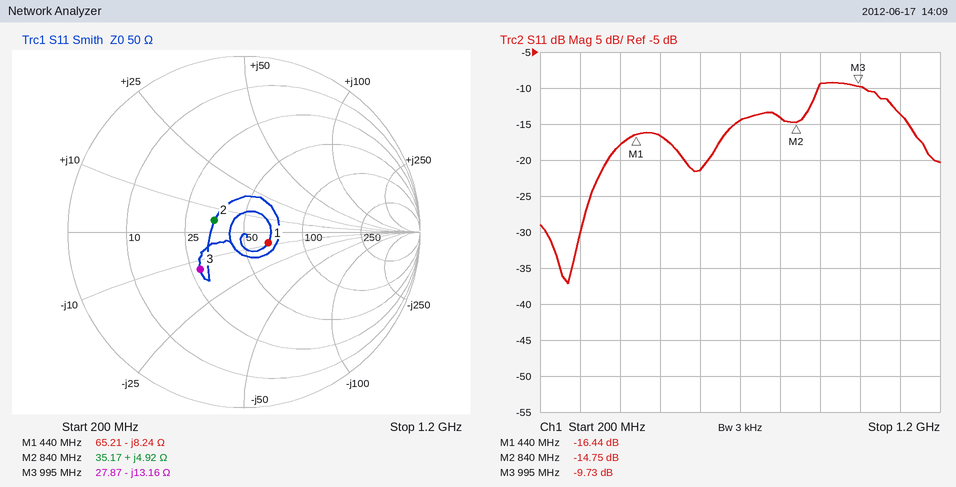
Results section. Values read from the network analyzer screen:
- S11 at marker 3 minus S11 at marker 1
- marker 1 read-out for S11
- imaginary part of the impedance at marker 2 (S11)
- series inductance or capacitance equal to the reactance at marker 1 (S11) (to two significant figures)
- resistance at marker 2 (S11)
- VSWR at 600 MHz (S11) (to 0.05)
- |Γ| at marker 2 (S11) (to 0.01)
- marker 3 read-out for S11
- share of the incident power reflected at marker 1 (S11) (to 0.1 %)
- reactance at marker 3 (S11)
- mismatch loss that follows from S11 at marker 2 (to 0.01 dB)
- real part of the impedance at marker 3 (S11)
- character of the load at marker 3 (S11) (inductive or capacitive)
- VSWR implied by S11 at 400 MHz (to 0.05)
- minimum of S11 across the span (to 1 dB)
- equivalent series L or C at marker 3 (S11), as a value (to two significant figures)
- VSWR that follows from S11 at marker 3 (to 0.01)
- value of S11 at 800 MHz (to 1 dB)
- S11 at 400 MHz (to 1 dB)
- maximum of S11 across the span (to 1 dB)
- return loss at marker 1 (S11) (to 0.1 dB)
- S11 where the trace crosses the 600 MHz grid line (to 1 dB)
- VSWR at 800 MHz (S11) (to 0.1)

6.71 dB
-16.44 dB
+4.92 Ω
44 pF
35.17 Ω
1.20
0.18
-9.73 dB
2.3 %
-13.16 Ω
0.15 dB
27.87 Ω
capacitive
1.30
-37 dB
12 pF
1.97
-14 dB
-18 dB
-9 dB
16.5 dB
-21 dB
1.5
